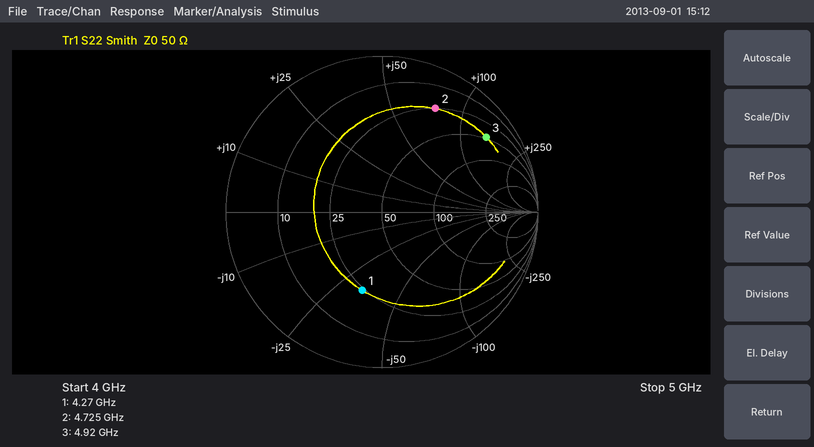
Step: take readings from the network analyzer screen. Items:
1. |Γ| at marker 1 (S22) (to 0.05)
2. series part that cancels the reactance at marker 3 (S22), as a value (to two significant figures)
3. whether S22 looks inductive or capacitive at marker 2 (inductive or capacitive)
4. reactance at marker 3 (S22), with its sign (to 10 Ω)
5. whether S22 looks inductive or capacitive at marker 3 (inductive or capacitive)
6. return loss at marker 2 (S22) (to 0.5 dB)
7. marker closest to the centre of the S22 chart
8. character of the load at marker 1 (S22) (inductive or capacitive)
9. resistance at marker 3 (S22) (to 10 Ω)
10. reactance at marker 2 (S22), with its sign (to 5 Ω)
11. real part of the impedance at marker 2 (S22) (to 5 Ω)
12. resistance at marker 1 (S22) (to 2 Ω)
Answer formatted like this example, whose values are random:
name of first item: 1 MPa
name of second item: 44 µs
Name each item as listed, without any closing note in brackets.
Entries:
|Γ| at marker 1 (S22): 0.50
series part that cancels the reactance at marker 3 (S22), as a value: 230 fF
whether S22 looks inductive or capacitive at marker 2: inductive
reactance at marker 3 (S22), with its sign: +140 Ω
whether S22 looks inductive or capacitive at marker 3: inductive
return loss at marker 2 (S22): 2.5 dB
marker closest to the centre of the S22 chart: marker 1
character of the load at marker 1 (S22): capacitive
resistance at marker 3 (S22): 50 Ω
reactance at marker 2 (S22), with its sign: +75 Ω
real part of the impedance at marker 2 (S22): 25 Ω
resistance at marker 1 (S22): 24 Ω
